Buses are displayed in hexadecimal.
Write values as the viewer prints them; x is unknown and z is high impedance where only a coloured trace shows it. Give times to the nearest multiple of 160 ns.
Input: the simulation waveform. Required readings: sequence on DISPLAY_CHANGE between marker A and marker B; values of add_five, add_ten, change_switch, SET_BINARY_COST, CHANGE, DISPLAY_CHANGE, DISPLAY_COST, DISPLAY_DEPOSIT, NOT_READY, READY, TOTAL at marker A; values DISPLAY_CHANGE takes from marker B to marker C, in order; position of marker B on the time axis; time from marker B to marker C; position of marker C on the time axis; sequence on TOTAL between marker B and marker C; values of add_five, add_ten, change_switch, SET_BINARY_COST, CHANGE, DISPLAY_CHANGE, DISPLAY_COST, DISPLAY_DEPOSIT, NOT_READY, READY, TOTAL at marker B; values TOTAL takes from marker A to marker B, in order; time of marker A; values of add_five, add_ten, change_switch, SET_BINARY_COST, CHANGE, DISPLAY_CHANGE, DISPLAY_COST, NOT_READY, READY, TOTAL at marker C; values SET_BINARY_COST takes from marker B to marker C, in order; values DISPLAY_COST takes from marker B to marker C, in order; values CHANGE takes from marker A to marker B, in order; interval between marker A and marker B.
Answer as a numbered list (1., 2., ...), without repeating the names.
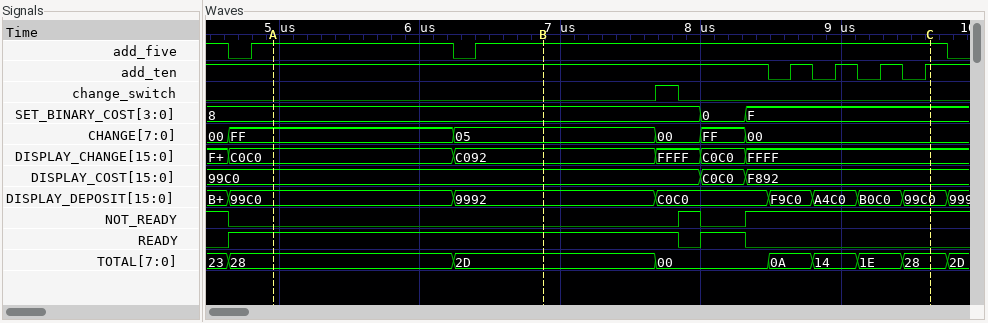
1. C0C0, C092
2. add_five=1, add_ten=1, change_switch=0, SET_BINARY_COST=8, CHANGE=FF, DISPLAY_CHANGE=C0C0, DISPLAY_COST=99C0, DISPLAY_DEPOSIT=99C0, NOT_READY=0, READY=1, TOTAL=28
3. C092, FFFF, C0C0, FFFF
4. 6880 ns
5. 2720 ns
6. 9600 ns
7. 2D, 00, 0A, 14, 1E, 28
8. add_five=1, add_ten=1, change_switch=0, SET_BINARY_COST=8, CHANGE=05, DISPLAY_CHANGE=C092, DISPLAY_COST=99C0, DISPLAY_DEPOSIT=9992, NOT_READY=0, READY=1, TOTAL=2D
9. 28, 2D
10. 4960 ns
11. add_five=1, add_ten=1, change_switch=0, SET_BINARY_COST=F, CHANGE=00, DISPLAY_CHANGE=FFFF, DISPLAY_COST=F892, NOT_READY=1, READY=0, TOTAL=28
12. 8, 0, F
13. 99C0, C0C0, F892
14. FF, 05
15. 1920 ns
